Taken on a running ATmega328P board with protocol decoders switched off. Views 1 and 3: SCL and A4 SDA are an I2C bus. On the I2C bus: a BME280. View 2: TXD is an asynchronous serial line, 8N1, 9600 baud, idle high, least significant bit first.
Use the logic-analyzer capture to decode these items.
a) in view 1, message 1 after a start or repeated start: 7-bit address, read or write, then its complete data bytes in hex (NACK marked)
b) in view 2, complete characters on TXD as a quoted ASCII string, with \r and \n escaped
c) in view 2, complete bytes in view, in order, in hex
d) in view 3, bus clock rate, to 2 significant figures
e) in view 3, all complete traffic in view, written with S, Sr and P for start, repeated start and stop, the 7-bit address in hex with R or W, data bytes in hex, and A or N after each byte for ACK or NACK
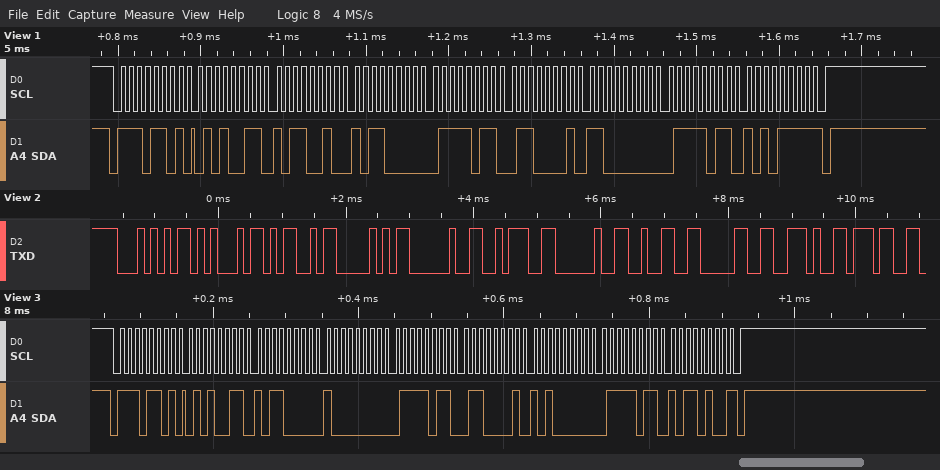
0x76 read: 53 B2 B0 7B 61 C0 7B AF NACK
"TEMP : 20.7"
54 45 4D 50 20 3A 20 32 30 2E 37
100 kHz
S 76R A 53 A B0 A 80 A 7B A 61 A A0 A 7B A B4 N P
